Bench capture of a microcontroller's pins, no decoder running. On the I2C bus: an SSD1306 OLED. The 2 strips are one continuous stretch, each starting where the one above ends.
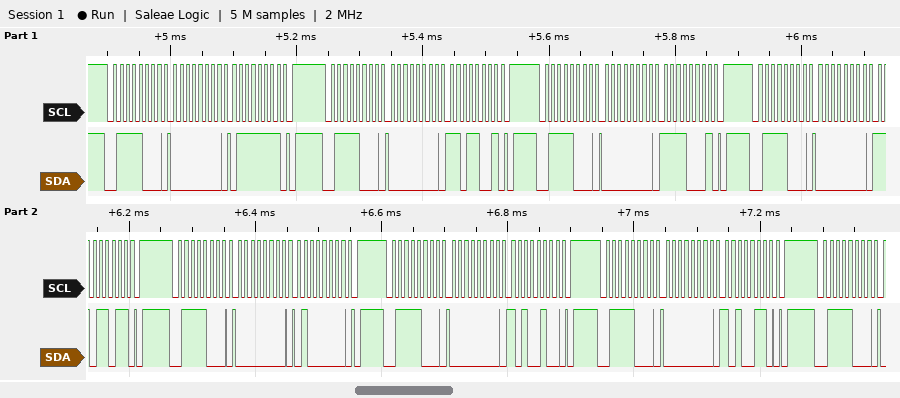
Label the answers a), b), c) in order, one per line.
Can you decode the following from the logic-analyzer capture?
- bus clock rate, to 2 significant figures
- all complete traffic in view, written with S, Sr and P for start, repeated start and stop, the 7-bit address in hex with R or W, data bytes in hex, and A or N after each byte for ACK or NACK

a) 100 kHz
b) S 3CW A 00 A 7F A P S 3CW A 00 A D9 A P S 3CW A 00 A F1 A P S 3CW A 00 A DB A P S 3CW A 00 A 40 A P S 3CW A 00 A A4 A P S 3CW A 00 A A6 A P S 3CW A
